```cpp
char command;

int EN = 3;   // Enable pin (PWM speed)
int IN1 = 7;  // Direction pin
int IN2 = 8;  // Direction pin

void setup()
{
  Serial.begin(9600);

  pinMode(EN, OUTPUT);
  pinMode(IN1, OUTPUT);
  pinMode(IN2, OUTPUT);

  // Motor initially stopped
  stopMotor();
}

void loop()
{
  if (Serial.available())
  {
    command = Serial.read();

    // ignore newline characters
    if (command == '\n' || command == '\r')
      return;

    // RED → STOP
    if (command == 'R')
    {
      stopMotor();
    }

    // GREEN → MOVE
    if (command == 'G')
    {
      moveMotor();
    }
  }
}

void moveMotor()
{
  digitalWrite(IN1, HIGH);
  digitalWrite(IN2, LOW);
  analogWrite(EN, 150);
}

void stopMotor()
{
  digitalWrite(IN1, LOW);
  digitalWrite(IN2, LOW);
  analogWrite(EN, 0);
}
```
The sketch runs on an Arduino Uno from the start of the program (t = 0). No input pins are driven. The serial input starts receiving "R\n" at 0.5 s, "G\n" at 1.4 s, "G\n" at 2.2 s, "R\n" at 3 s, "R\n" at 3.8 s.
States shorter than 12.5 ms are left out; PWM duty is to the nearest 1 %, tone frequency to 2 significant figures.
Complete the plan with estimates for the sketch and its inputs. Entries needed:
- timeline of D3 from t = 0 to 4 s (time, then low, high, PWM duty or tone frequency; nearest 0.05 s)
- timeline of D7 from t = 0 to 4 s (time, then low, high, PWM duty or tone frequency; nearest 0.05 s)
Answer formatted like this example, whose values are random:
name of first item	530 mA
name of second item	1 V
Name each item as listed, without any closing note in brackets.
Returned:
timeline of D3 from t = 0 to 4 s	0 s low; 1.4 s PWM 59 %; 3 s low
timeline of D7 from t = 0 to 4 s	0 s low; 1.4 s high; 3 s low
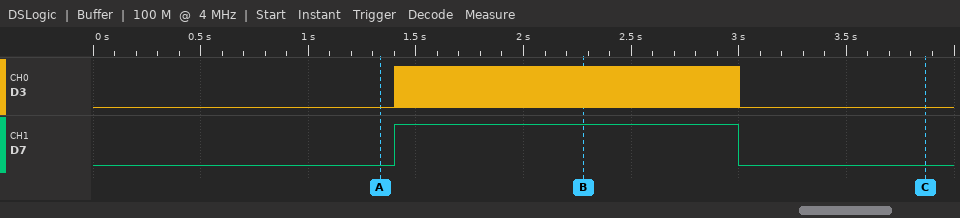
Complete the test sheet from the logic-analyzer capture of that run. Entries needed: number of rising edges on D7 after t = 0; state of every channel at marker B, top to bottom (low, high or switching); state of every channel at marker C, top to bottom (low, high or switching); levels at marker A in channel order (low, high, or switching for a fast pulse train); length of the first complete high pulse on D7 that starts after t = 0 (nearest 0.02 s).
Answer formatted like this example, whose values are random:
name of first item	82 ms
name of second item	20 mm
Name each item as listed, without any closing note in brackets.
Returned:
number of rising edges on D7 after t = 0	1
state of every channel at marker B, top to bottom	D3 switching, D7 high
state of every channel at marker C, top to bottom	D3 low, D7 low
levels at marker A in channel order	D3 low, D7 low
length of the first complete high pulse on D7 that starts after t = 0	1.60 s
